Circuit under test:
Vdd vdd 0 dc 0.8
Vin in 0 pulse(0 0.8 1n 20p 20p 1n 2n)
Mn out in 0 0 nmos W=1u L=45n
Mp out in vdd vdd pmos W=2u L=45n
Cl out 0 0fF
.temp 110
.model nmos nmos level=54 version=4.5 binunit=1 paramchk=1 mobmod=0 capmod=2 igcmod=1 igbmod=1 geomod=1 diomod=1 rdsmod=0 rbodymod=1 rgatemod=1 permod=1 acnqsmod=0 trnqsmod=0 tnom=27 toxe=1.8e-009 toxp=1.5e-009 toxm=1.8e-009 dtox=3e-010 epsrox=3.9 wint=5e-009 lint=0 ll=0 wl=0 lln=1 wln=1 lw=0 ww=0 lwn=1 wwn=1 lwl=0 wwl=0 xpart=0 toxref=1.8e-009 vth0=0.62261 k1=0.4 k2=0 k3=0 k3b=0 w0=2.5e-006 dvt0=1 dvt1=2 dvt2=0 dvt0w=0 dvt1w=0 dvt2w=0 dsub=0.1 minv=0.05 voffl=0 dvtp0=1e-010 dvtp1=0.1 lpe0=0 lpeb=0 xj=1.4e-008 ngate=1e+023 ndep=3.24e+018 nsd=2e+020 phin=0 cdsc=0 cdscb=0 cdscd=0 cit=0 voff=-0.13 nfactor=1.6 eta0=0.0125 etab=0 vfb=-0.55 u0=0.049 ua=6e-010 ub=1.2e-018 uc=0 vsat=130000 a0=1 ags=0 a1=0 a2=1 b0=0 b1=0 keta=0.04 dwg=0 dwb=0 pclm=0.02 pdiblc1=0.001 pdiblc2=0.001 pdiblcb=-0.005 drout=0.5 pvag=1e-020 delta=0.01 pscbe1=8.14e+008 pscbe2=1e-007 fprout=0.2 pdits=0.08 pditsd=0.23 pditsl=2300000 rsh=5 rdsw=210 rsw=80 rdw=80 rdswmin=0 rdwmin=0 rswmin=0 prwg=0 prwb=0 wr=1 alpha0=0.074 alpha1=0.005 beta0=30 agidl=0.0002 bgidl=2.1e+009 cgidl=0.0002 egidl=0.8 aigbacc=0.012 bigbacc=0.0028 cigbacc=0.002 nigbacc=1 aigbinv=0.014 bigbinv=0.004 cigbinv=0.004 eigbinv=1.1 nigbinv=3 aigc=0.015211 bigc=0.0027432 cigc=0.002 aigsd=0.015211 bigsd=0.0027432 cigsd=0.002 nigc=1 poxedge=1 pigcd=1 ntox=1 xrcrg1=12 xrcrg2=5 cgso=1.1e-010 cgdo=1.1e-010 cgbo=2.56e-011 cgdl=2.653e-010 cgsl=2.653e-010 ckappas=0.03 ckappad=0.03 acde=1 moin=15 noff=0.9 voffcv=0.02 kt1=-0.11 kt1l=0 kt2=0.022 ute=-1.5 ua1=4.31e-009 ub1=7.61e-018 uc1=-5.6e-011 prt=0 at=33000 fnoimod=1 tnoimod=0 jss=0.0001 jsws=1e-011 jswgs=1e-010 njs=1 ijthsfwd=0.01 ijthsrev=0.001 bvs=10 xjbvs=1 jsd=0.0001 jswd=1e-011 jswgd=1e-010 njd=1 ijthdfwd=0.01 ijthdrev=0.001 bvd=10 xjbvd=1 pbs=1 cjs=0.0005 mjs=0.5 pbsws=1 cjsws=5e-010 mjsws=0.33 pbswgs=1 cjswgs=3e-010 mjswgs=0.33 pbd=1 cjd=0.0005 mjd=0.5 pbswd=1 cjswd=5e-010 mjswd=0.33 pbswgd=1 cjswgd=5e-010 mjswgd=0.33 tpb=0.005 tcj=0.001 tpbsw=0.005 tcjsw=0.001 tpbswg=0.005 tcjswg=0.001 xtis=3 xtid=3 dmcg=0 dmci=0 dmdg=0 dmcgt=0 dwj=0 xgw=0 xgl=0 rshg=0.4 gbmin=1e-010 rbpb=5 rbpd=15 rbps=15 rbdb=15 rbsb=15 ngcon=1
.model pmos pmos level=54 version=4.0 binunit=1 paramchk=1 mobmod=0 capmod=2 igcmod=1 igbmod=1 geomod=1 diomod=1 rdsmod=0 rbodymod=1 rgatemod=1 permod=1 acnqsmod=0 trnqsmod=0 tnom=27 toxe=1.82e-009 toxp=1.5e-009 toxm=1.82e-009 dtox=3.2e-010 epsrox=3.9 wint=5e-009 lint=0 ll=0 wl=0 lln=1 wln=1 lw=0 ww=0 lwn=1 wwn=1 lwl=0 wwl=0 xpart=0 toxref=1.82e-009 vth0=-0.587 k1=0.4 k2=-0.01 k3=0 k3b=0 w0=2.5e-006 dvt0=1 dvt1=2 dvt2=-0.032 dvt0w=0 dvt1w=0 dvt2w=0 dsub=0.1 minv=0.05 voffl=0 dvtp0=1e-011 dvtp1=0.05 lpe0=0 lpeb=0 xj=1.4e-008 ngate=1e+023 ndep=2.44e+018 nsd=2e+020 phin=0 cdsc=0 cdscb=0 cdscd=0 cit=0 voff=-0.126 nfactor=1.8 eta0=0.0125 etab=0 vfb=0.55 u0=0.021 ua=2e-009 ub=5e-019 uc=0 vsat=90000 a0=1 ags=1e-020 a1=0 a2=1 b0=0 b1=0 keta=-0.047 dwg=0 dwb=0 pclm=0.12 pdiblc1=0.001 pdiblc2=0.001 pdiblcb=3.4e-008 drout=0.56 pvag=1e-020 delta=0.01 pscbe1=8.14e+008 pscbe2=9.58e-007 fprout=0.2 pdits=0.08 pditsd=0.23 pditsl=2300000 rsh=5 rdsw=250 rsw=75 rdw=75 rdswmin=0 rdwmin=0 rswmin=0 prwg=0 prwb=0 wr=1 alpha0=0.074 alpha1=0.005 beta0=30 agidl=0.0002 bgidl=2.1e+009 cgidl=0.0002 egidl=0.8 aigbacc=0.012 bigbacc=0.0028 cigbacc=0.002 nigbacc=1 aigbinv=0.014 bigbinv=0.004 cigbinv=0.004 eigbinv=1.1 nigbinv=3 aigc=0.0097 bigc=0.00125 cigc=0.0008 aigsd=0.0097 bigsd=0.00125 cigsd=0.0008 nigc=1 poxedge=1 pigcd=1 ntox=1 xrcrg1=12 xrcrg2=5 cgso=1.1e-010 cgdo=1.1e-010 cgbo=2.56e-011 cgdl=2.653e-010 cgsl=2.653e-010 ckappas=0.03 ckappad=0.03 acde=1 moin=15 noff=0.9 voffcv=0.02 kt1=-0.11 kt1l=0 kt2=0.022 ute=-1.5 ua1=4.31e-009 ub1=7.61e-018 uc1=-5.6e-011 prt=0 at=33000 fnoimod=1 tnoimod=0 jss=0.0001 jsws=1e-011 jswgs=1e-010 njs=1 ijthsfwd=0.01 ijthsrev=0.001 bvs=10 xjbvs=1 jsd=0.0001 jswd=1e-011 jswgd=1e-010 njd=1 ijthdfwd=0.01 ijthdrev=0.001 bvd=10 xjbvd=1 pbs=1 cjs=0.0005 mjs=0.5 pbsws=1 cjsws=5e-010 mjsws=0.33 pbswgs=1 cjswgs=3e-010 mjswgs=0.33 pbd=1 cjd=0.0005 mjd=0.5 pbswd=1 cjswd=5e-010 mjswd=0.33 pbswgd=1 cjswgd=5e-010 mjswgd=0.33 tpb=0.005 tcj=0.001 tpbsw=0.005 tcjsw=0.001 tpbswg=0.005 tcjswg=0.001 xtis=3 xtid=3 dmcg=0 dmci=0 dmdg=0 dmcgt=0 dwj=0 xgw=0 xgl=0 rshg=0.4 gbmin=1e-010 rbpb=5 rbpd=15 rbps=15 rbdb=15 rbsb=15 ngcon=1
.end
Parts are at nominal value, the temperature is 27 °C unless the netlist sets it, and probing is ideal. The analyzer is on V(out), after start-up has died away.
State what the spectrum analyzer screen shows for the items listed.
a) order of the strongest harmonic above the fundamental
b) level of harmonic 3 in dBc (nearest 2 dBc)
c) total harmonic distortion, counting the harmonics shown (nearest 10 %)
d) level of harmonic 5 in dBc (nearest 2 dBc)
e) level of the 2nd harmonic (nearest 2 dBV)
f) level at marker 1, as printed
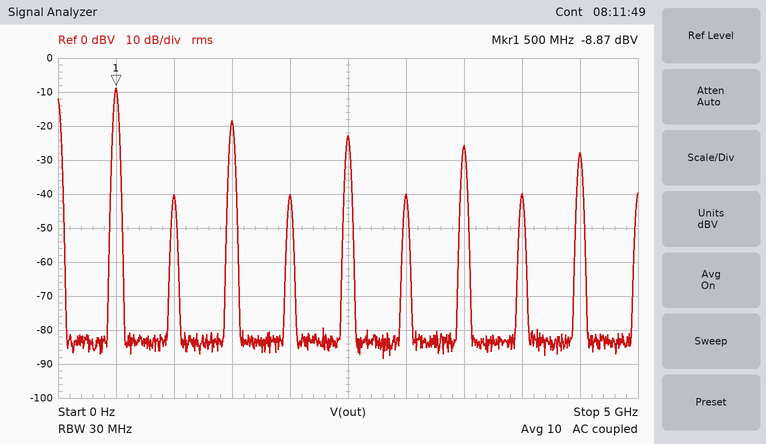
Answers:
3
-10 dBc
40 %
-14 dBc
-40 dBV
-8.87 dBV
